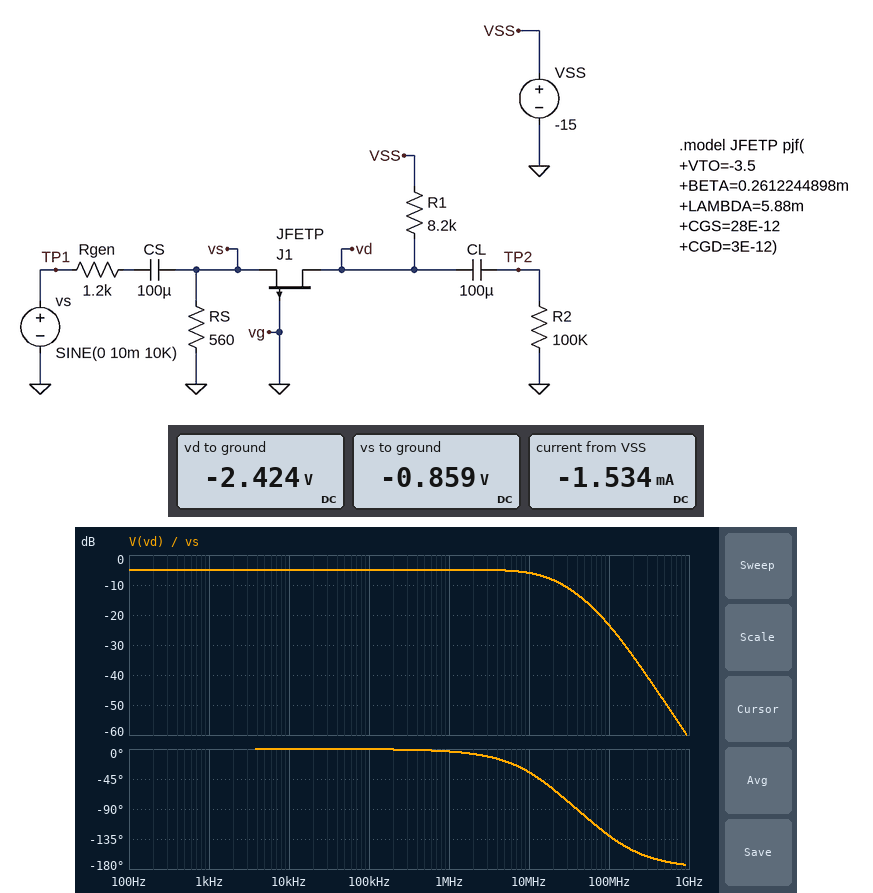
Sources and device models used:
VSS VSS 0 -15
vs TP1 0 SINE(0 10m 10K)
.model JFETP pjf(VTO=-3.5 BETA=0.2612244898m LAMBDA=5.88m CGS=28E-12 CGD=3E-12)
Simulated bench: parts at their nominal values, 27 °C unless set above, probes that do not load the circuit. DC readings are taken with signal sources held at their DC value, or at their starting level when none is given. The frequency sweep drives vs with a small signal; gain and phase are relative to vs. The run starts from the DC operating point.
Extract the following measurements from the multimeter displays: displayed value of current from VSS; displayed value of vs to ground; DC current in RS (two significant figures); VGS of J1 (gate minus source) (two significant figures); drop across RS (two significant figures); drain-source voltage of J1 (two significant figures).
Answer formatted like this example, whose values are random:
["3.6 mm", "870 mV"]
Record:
["-1.534 mA", "-0.859 V", "1.5 mA", "860 mV", "860 mV", "-1.6 V"]
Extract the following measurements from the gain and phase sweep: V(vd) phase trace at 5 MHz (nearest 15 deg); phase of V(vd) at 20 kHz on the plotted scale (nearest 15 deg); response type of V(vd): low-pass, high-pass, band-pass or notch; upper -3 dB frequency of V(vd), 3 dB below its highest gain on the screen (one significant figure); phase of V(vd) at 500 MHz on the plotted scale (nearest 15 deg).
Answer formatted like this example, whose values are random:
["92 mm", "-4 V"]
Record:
["-15 deg", "0 deg", "low-pass", "20 MHz", "-165 deg"]
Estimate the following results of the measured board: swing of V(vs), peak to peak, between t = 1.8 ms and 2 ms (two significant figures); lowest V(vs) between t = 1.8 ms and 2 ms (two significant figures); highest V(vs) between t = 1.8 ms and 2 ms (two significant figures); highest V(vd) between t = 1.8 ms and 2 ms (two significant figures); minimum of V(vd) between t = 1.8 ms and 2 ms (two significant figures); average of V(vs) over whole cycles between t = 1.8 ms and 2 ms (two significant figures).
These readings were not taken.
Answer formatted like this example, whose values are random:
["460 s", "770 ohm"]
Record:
["5.8 mV", "-860 mV", "-860 mV", "-2.4 V", "-2.4 V", "-860 mV"]
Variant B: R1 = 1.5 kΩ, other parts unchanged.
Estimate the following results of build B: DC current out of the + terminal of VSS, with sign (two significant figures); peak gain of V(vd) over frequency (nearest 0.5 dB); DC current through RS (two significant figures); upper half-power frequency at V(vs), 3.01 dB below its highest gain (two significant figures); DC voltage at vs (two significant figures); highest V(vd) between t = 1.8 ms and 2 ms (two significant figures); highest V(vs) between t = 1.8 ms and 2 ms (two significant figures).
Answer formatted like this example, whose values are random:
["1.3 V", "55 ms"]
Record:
["-1.8 mA", "-7.5 dB", "1.8 mA", "32 MHz", "-990 mV", "-12 V", "-980 mV"]
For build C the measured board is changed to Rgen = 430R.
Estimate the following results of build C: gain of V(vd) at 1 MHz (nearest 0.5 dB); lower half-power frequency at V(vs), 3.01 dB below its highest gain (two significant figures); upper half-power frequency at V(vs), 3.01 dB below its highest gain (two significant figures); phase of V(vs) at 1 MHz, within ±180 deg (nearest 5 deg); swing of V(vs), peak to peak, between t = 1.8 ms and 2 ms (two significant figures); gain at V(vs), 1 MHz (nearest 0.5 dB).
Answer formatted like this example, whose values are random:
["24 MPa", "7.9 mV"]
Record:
["0.5 dB", "1.7 Hz", "29 MHz", "0 deg", "11 mV", "-5.5 dB"]
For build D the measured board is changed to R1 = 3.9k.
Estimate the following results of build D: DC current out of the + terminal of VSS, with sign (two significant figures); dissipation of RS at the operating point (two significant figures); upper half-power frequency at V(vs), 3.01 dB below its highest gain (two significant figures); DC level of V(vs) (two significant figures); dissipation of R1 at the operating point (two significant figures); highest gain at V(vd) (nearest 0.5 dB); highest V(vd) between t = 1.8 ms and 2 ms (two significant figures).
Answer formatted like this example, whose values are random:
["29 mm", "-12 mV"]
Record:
["-1.7 mA", "1.7 mW", "31 MHz", "-970 mV", "12 mW", "0.5 dB", "-8.2 V"]
